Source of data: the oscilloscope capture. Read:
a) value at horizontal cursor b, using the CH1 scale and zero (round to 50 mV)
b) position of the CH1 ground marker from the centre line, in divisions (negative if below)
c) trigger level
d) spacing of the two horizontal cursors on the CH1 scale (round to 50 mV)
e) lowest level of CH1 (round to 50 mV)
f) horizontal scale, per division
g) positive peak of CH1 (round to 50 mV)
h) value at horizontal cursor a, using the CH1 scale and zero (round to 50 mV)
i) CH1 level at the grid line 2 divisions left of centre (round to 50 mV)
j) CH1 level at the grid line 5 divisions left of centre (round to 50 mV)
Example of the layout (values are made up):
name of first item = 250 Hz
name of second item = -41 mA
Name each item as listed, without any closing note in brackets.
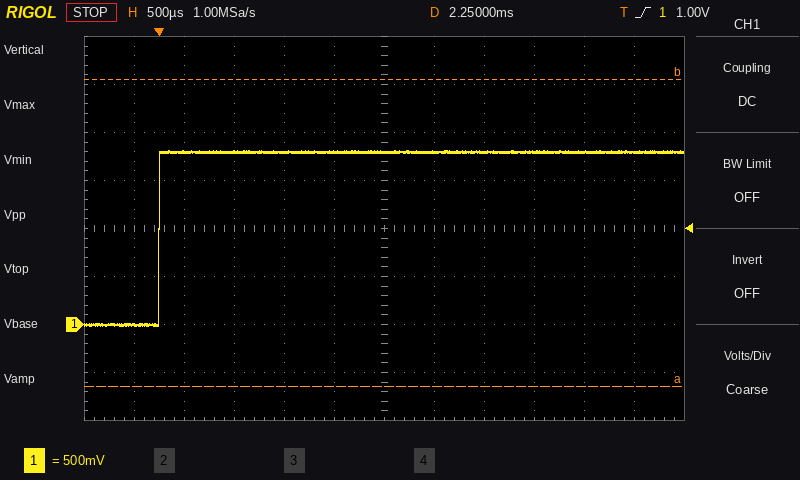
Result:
value at horizontal cursor b, using the CH1 scale and zero = 2.55 V
position of the CH1 ground marker from the centre line, in divisions = -2.0 div
trigger level = 1.00 V
spacing of the two horizontal cursors on the CH1 scale = 3.20 V
lowest level of CH1 = 0 mV
horizontal scale, per division = 500 µs
positive peak of CH1 = 1.80 V
value at horizontal cursor a, using the CH1 scale and zero = -650 mV
CH1 level at the grid line 2 divisions left of centre = 1.80 V
CH1 level at the grid line 5 divisions left of centre = 0 mV
